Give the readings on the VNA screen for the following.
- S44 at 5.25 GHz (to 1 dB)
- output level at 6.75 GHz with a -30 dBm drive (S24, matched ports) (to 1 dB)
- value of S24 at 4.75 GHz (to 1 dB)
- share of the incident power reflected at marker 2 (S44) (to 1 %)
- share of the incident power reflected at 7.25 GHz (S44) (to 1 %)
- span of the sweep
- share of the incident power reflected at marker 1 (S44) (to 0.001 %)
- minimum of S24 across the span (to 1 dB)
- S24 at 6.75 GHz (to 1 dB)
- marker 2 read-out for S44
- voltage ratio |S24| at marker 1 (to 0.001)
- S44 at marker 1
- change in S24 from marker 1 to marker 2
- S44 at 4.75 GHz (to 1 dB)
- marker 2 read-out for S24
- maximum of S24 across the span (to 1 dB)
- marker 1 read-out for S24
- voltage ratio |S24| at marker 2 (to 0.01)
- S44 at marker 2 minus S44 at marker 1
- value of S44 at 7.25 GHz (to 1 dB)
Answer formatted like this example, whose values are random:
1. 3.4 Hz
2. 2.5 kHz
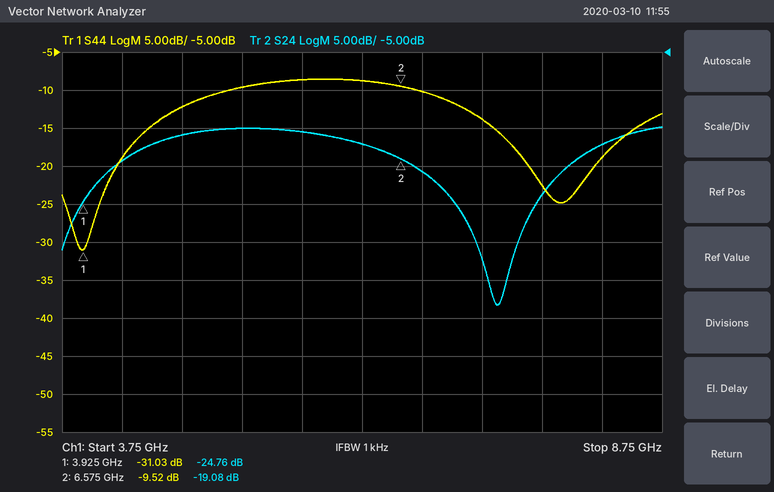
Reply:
1. -10 dB
2. -51 dBm
3. -16 dB
4. 11 %
5. 4 %
6. 5 GHz
7. 0.079 %
8. -38 dB
9. -21 dB
10. -9.52 dB
11. 0.058
12. -31.03 dB
13. 5.68 dB
14. -12 dB
15. -19.08 dB
16. -15 dB
17. -24.76 dB
18. 0.11
19. 21.51 dB
20. -14 dB
